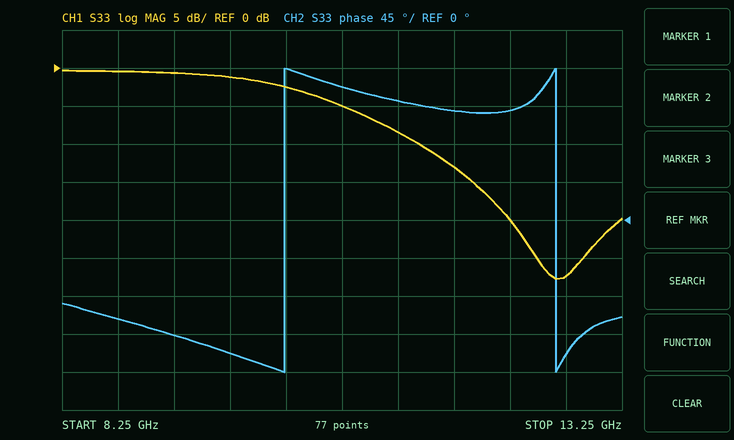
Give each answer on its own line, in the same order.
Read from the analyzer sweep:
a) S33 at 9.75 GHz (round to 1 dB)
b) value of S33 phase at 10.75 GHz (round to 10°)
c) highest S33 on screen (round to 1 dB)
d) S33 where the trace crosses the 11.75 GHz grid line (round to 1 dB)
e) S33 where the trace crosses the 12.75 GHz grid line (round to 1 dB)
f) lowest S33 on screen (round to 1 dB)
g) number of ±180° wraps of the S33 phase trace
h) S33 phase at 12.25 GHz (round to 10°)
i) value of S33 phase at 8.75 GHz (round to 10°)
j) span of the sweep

-1 dB
160°
0 dB
-13 dB
-27 dB
-28 dB
2
130°
-120°
5 GHz
